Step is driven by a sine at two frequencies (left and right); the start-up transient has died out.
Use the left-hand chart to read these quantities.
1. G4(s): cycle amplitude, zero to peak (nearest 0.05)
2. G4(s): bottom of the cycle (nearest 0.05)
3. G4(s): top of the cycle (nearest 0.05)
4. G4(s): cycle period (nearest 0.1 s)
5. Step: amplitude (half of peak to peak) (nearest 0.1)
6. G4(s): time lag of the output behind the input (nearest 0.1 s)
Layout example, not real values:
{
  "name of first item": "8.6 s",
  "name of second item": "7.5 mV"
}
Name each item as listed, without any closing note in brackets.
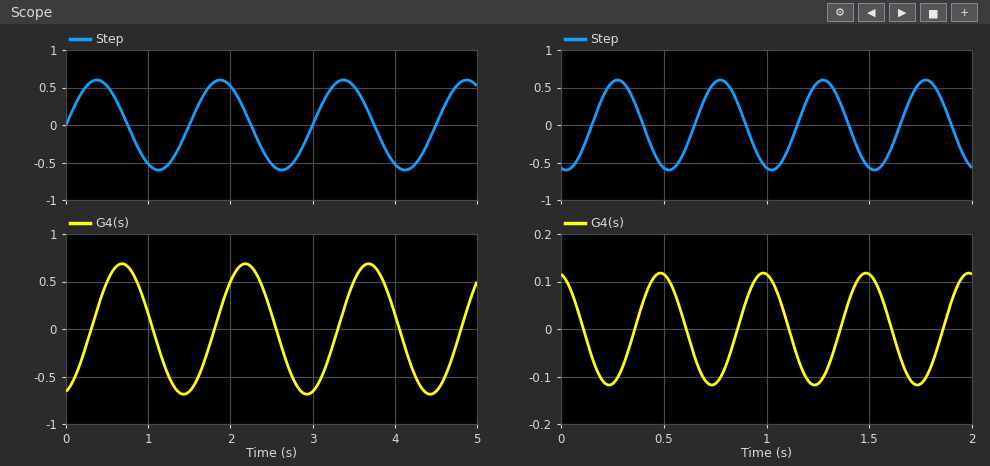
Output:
{
  "G4(s): cycle amplitude, zero to peak": "0.70",
  "G4(s): bottom of the cycle": "-0.70",
  "G4(s): top of the cycle": "0.70",
  "G4(s): cycle period": "1.5 s",
  "Step: amplitude (half of peak to peak)": "0.6",
  "G4(s): time lag of the output behind the input": "0.3 s"
}
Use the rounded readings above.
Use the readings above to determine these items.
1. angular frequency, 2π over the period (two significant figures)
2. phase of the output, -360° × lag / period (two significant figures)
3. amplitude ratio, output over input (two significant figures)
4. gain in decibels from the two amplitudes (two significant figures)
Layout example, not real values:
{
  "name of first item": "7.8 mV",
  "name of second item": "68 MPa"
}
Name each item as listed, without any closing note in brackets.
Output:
{
  "angular frequency, 2π over the period": "4.2 rad/s",
  "phase of the output, -360° × lag / period": "-72°",
  "amplitude ratio, output over input": "1.2",
  "gain in decibels from the two amplitudes": "1.3 dB"
}
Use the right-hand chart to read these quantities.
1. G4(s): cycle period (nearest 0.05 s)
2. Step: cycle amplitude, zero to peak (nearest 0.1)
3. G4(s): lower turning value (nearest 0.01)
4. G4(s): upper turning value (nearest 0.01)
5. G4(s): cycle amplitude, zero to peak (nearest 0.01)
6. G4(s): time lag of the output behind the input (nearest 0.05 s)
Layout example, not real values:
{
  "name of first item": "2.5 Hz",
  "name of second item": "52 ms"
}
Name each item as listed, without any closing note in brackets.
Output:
{
  "G4(s): cycle period": "0.50 s",
  "Step: cycle amplitude, zero to peak": "0.6",
  "G4(s): lower turning value": "-0.12",
  "G4(s): upper turning value": "0.12",
  "G4(s): cycle amplitude, zero to peak": "0.12",
  "G4(s): time lag of the output behind the input": "0.20 s"
}
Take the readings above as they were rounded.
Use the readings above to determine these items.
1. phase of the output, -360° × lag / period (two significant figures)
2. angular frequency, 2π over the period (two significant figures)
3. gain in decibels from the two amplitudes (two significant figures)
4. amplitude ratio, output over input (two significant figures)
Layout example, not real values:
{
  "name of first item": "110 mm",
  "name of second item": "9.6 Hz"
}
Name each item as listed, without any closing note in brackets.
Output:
{
  "phase of the output, -360° × lag / period": "-140°",
  "angular frequency, 2π over the period": "13 rad/s",
  "gain in decibels from the two amplitudes": "-14 dB",
  "amplitude ratio, output over input": "0.20"
}
